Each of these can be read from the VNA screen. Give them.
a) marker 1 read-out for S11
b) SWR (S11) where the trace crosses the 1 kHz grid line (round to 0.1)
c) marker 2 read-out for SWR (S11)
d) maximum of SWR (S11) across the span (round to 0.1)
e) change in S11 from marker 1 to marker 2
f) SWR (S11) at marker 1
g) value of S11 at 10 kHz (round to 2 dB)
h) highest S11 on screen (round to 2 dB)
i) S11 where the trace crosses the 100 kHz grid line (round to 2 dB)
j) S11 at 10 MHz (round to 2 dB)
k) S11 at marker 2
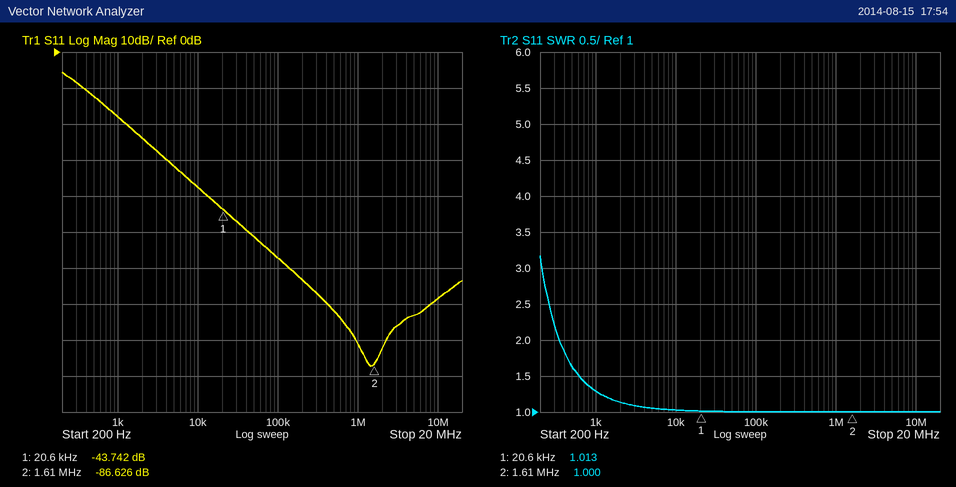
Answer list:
-43.742 dB
1.3
1.000
3.2
-42.884 dB
1.013
-38 dB
-6 dB
-58 dB
-68 dB
-86.626 dB
